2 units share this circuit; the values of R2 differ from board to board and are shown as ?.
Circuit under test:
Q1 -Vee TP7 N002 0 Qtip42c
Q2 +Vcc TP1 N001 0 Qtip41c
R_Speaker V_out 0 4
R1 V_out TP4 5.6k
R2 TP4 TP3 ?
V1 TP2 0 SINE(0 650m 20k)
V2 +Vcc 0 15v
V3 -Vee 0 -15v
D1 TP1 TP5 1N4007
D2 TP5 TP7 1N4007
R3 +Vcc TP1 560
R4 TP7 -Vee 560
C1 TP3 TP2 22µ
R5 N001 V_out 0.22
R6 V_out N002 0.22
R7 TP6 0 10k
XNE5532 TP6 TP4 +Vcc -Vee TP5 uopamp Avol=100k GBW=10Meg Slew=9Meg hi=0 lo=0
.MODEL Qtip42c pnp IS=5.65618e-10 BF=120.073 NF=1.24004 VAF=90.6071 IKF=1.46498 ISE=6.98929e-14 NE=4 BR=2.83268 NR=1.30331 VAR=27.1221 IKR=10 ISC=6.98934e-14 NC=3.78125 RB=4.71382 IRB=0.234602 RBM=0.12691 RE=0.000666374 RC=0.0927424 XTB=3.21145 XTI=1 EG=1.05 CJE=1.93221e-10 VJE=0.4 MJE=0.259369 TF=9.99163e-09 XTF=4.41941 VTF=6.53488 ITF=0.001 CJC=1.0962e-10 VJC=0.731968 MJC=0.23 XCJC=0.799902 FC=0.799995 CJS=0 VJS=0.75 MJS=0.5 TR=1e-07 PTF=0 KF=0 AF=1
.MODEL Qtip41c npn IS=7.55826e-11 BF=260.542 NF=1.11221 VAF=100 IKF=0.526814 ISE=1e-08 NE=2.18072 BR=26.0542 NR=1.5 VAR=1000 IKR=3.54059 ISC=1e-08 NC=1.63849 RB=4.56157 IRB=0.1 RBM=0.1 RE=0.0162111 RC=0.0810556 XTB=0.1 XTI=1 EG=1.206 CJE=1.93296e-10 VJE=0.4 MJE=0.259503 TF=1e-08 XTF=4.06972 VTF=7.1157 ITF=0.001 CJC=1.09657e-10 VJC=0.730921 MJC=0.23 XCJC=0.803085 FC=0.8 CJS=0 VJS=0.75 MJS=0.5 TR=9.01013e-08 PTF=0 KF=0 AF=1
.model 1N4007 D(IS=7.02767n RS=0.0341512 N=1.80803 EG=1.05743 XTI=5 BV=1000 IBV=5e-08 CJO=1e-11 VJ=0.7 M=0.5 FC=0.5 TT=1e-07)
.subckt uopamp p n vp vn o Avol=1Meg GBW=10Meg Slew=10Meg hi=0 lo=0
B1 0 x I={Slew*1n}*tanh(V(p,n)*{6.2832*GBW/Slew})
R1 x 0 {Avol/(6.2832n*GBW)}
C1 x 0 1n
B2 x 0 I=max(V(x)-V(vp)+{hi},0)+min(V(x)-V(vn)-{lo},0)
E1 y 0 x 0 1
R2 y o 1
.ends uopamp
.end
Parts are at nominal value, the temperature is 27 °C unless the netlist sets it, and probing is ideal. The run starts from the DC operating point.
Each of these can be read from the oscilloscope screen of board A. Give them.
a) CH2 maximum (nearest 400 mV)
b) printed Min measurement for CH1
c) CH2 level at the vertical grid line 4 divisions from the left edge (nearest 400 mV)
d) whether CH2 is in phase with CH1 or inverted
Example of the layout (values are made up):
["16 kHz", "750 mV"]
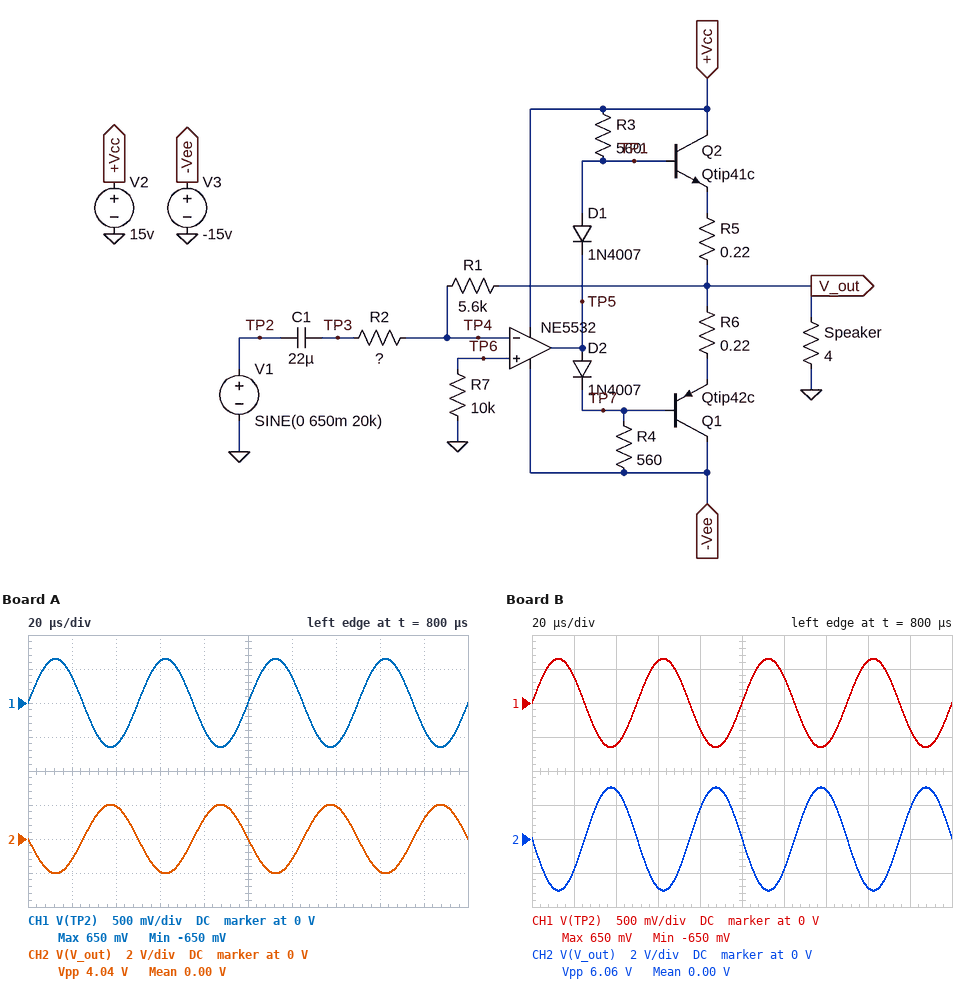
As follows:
["2.0 V", "-650 mV", "1.2 V", "inverted"]
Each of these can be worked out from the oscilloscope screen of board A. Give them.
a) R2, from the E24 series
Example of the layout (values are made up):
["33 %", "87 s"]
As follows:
["1.8 kΩ"]
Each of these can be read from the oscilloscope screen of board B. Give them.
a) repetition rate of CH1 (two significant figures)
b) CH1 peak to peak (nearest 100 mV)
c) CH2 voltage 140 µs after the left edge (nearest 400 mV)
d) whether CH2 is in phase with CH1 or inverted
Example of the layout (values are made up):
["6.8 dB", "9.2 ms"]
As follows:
["20 kHz", "1.3 V", "2.8 V", "inverted"]
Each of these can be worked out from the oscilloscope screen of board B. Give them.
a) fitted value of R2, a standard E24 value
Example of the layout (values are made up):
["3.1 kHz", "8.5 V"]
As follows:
["1.2 kΩ"]
